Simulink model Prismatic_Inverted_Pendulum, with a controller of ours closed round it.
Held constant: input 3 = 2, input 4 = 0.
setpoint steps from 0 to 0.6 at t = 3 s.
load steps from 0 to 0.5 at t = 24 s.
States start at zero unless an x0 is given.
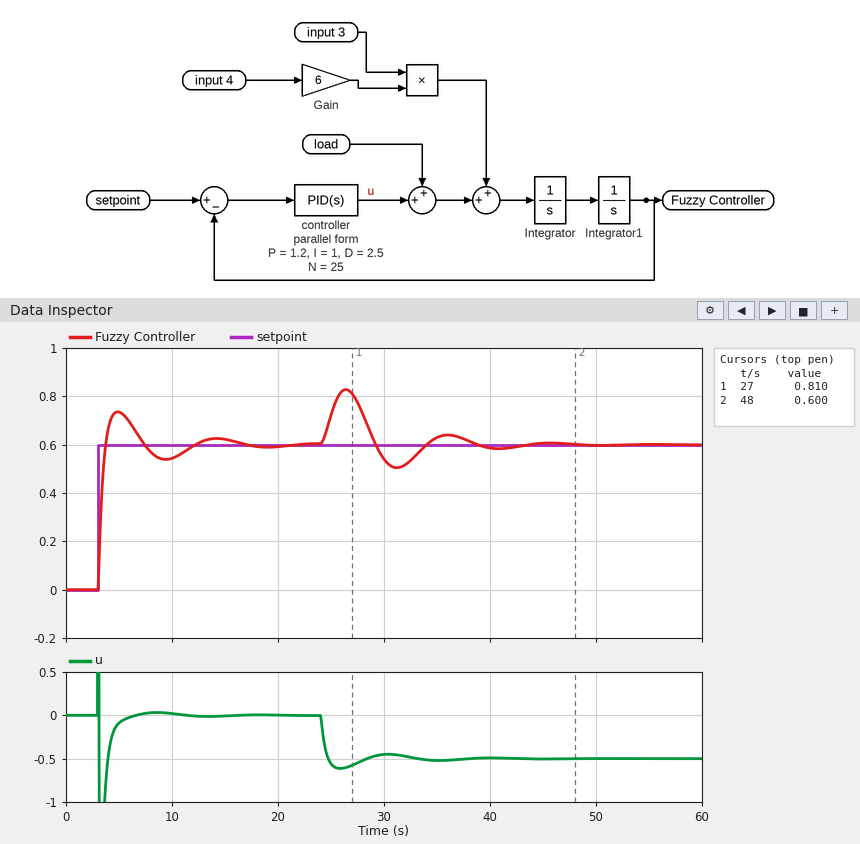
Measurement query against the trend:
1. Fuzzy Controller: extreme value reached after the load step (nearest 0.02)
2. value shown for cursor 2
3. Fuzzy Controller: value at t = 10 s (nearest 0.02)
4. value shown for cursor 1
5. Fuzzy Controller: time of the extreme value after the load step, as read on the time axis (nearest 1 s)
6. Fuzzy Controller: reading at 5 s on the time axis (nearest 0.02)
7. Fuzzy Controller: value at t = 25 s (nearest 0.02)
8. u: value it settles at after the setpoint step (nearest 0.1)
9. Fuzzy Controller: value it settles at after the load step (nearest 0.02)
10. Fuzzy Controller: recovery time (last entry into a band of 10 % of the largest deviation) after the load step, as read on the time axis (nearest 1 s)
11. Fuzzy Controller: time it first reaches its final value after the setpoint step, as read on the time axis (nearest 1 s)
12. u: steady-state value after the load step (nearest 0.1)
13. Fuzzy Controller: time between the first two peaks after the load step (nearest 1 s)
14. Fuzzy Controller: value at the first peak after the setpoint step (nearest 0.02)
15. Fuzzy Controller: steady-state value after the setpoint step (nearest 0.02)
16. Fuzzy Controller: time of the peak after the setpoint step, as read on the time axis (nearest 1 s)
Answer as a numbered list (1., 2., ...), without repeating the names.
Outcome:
1. 0.82
2. 0.600
3. 0.54
4. 0.810
5. 26 s
6. 0.74
7. 0.72
8. 0.0
9. 0.60
10. 38 s
11. 4 s
12. -0.5
13. 10 s
14. 0.74
15. 0.60
16. 5 s
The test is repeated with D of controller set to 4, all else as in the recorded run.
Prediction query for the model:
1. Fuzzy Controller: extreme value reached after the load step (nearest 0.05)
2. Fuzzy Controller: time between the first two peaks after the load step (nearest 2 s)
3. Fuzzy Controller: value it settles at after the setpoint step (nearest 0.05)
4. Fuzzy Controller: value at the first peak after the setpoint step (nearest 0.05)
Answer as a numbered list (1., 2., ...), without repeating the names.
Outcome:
1. 0.80
2. 12 s
3. 0.60
4. 0.65
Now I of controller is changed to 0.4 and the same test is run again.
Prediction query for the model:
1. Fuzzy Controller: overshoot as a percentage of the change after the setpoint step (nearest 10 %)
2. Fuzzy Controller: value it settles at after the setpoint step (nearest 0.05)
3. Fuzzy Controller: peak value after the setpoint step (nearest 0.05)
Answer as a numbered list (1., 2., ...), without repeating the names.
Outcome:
1. 20 %
2. 0.60
3. 0.70
